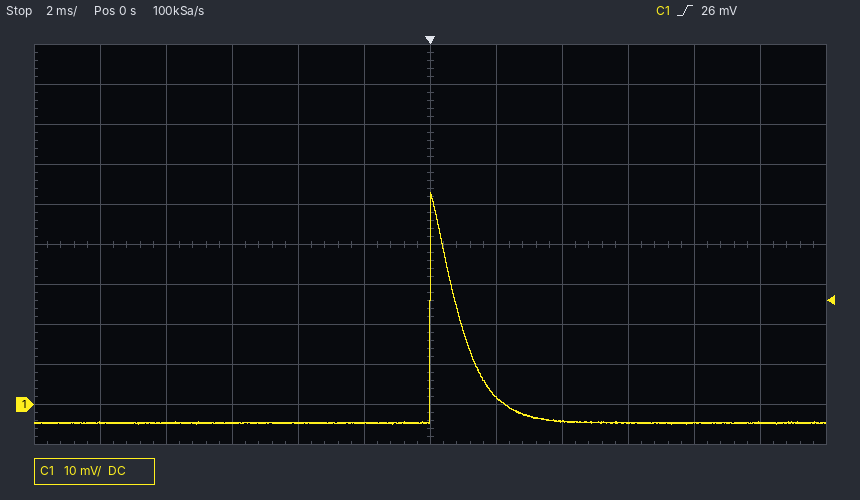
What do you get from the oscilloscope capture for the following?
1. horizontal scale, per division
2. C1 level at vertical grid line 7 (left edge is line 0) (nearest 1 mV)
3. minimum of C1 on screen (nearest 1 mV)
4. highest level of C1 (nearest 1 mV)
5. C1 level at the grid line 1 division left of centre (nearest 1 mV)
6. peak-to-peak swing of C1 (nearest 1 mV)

2 ms
2 mV
-5 mV
53 mV
-5 mV
58 mV
